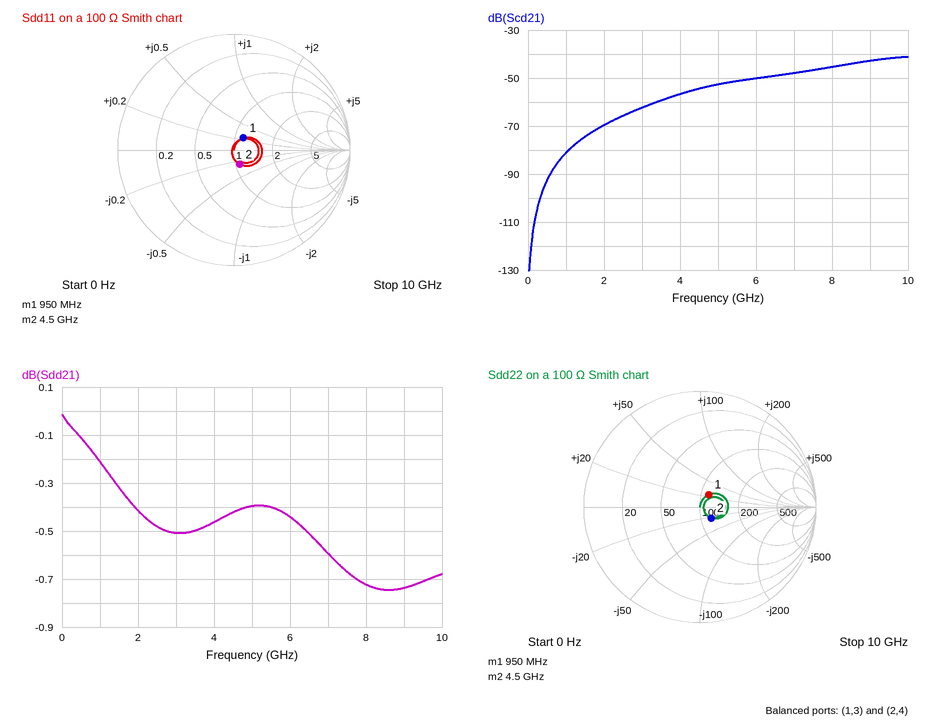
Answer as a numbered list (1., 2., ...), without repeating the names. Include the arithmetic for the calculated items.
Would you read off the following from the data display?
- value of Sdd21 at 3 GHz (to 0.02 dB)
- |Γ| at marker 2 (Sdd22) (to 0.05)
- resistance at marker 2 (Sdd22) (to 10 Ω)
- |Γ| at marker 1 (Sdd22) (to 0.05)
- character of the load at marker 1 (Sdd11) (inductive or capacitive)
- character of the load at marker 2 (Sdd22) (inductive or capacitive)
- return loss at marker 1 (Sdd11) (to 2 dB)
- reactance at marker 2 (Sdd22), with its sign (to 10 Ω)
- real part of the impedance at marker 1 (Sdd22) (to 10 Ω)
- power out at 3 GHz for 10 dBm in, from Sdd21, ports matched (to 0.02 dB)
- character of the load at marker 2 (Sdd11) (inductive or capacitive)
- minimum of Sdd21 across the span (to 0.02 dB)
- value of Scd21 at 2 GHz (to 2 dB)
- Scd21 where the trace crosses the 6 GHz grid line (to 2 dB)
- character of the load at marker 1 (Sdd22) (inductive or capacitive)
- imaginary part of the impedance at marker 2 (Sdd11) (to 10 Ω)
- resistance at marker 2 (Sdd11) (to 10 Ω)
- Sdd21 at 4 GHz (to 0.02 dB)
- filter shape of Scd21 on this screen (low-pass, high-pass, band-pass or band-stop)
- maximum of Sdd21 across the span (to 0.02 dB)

1. -0.50 dB
2. 0.15
3. 120 Ω
4. 0.15
5. inductive
6. capacitive
7. 18 dB
8. -20 Ω
9. 110 Ω
10. 10 dBm + (-0.50 dB) = 9.50 dBm
11. capacitive
12. -0.74 dB
13. -70 dB
14. -50 dB
15. inductive
16. -30 Ω
17. 110 Ω
18. -0.46 dB
19. high-pass
20. -0.02 dB
